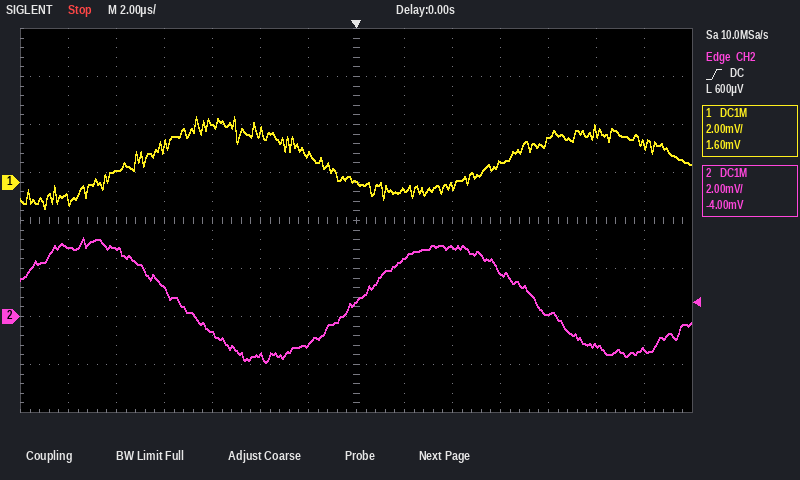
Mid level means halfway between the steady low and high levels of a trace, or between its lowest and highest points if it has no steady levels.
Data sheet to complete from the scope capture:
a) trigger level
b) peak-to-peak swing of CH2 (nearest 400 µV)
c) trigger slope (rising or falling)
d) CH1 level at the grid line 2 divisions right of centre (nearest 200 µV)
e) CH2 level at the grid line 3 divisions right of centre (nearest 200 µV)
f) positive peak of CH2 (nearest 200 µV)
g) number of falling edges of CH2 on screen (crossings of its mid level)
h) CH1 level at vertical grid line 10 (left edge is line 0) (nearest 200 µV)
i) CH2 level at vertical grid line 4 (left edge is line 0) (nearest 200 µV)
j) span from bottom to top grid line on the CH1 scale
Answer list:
600 µV
5.2 mV
rising
-200 µV
1.8 mV
3.2 mV
2
800 µV
-600 µV
16 mV
